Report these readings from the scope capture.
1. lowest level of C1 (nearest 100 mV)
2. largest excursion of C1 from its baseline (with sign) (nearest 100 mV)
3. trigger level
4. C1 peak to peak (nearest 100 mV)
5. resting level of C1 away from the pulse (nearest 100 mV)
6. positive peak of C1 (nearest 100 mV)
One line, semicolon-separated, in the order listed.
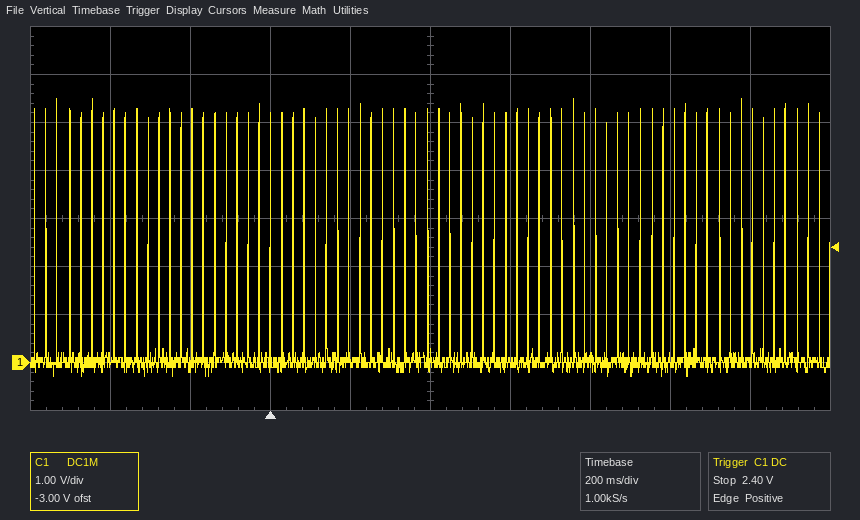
-300 mV; +5.5 V; 2.40 V; 5.8 V; 0.0 V; 5.5 V
